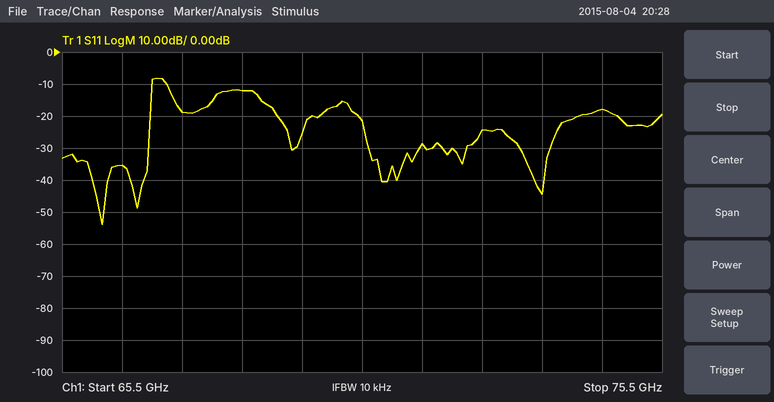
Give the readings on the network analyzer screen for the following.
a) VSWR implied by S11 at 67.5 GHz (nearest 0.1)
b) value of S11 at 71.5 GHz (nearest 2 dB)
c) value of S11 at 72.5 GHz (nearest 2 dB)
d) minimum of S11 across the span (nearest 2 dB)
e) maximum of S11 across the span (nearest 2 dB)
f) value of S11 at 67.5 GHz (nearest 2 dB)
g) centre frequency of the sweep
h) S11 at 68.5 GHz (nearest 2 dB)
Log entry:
1.3
-28 dB
-24 dB
-54 dB
-8 dB
-18 dB
70.5 GHz
-12 dB
